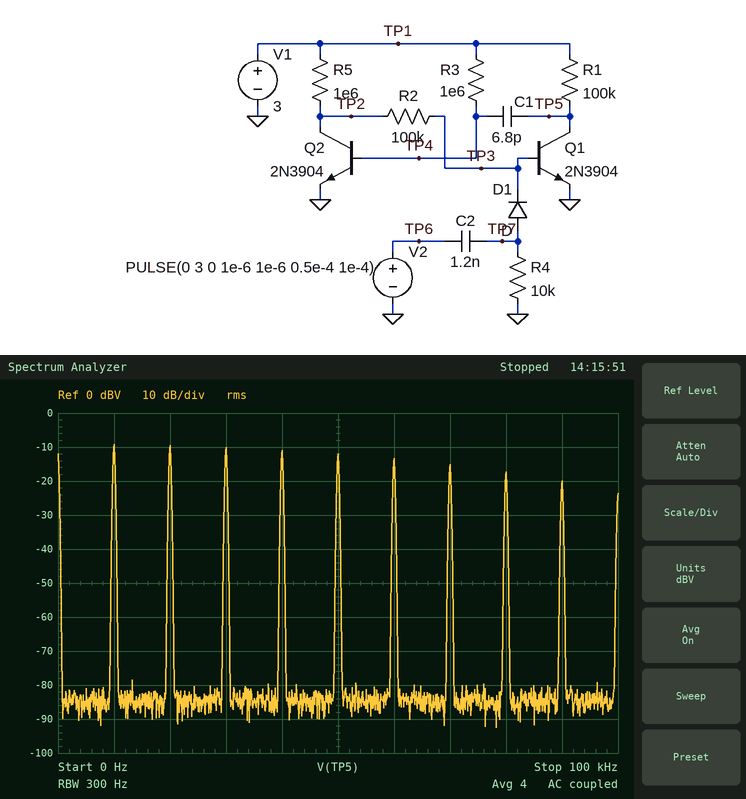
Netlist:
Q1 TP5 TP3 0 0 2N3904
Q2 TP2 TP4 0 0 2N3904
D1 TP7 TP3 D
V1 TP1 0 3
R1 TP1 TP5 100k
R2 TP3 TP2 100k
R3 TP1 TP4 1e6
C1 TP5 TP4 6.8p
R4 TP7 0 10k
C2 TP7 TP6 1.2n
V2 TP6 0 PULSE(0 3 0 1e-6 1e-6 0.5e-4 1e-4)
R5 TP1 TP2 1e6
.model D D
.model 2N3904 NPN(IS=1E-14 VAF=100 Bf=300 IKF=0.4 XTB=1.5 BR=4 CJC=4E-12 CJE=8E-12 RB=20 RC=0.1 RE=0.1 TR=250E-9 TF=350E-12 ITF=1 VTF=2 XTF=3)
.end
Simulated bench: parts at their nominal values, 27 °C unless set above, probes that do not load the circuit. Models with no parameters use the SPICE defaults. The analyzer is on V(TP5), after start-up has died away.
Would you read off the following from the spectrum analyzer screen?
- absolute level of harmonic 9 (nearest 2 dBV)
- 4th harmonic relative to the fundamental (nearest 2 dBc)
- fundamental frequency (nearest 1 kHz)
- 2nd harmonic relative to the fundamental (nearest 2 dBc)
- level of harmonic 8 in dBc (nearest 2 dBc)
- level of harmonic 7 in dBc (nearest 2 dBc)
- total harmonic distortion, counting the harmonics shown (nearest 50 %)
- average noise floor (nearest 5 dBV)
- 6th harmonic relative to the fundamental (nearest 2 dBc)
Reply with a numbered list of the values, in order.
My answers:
1. -20 dBV
2. -2 dBc
3. 10 kHz
4. 0 dBc
5. -8 dBc
6. -6 dBc
7. 200 %
8. -85 dBV
9. -4 dBc
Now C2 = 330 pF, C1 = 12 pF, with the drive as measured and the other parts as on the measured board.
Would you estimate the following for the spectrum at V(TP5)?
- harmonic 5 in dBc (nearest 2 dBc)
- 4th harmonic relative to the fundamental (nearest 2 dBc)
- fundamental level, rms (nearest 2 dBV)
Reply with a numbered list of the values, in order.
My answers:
1. -6 dBc
2. -4 dBc
3. -6 dBV
